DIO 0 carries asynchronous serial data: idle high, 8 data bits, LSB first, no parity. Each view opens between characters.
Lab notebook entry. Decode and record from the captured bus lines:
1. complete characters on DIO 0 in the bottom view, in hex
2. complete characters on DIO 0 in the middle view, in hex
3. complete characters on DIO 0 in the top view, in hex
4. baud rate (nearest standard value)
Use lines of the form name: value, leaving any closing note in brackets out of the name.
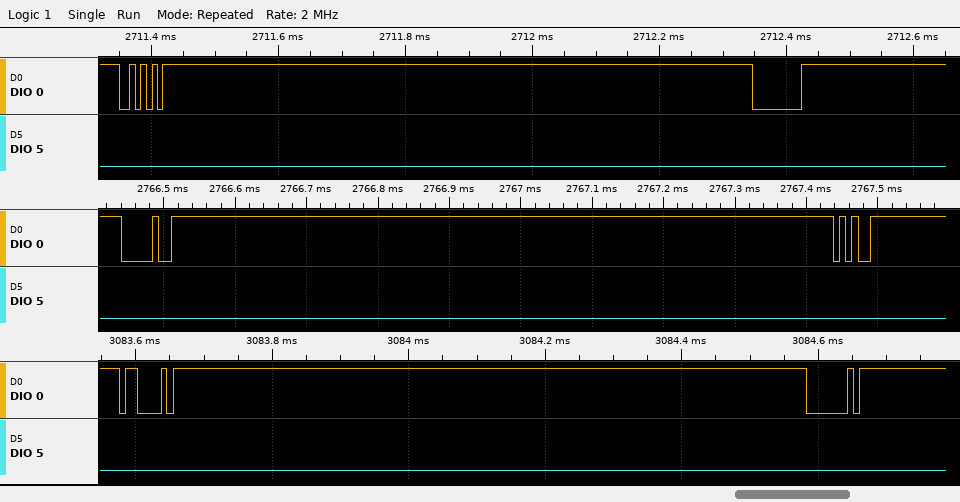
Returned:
complete characters on DIO 0 in the bottom view, in hex: 43, 40
complete characters on DIO 0 in the middle view, in hex: 90, E5
complete characters on DIO 0 in the top view, in hex: AA, 00
baud rate: 115200 baud
